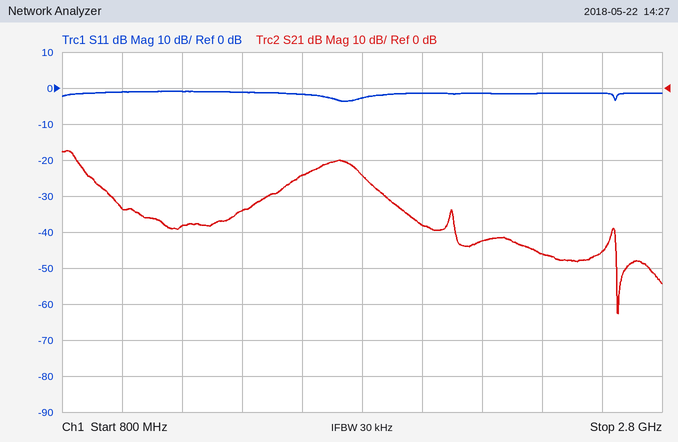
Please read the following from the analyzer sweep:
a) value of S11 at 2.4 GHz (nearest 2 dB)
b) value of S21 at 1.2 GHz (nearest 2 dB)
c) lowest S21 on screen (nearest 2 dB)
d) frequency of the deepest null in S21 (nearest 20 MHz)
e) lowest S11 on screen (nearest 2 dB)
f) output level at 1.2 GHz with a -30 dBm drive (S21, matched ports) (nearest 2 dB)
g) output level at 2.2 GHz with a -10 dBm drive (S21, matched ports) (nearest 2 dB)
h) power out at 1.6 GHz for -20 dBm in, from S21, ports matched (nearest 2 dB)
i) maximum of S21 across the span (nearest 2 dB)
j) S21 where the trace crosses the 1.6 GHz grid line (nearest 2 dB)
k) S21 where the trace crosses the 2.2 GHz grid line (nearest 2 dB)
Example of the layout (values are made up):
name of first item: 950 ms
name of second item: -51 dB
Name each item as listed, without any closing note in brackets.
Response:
value of S11 at 2.4 GHz: -2 dB
value of S21 at 1.2 GHz: -38 dB
lowest S21 on screen: -62 dB
frequency of the deepest null in S21: 2.66 GHz
lowest S11 on screen: -4 dB
output level at 1.2 GHz with a -30 dBm drive (S21, matched ports): -68 dBm
output level at 2.2 GHz with a -10 dBm drive (S21, matched ports): -52 dBm
power out at 1.6 GHz for -20 dBm in, from S21, ports matched: -44 dBm
maximum of S21 across the span: -18 dB
S21 where the trace crosses the 1.6 GHz grid line: -24 dB
S21 where the trace crosses the 2.2 GHz grid line: -42 dB
